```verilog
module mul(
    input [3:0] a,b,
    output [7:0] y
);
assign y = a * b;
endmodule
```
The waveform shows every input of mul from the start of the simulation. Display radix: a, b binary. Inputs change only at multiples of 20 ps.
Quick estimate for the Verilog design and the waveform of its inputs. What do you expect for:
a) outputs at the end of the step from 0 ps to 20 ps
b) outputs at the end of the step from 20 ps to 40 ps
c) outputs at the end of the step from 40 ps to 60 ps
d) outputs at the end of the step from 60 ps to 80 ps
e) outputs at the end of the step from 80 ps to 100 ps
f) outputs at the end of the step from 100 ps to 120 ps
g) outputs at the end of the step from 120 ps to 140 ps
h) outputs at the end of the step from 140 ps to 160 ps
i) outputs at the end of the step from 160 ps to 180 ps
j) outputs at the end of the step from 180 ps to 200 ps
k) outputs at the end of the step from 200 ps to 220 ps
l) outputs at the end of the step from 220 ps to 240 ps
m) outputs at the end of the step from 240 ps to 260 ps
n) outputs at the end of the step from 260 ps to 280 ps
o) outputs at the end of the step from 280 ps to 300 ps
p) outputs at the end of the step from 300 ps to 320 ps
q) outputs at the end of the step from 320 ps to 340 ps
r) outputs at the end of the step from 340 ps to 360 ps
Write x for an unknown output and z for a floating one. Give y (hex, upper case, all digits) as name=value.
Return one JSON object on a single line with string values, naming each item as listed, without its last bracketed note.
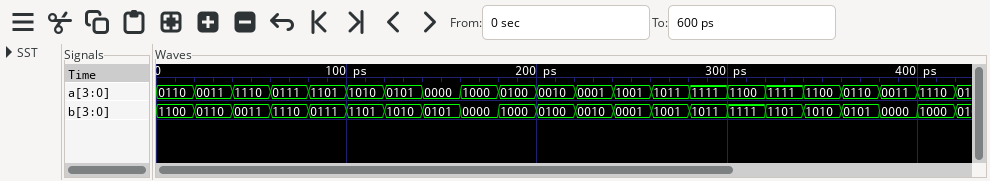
{"outputs at the end of the step from 0 ps to 20 ps": "y=48", "outputs at the end of the step from 20 ps to 40 ps": "y=12", "outputs at the end of the step from 40 ps to 60 ps": "y=2A", "outputs at the end of the step from 60 ps to 80 ps": "y=62", "outputs at the end of the step from 80 ps to 100 ps": "y=5B", "outputs at the end of the step from 100 ps to 120 ps": "y=82", "outputs at the end of the step from 120 ps to 140 ps": "y=32", "outputs at the end of the step from 140 ps to 160 ps": "y=00", "outputs at the end of the step from 160 ps to 180 ps": "y=00", "outputs at the end of the step from 180 ps to 200 ps": "y=20", "outputs at the end of the step from 200 ps to 220 ps": "y=08", "outputs at the end of the step from 220 ps to 240 ps": "y=02", "outputs at the end of the step from 240 ps to 260 ps": "y=09", "outputs at the end of the step from 260 ps to 280 ps": "y=63", "outputs at the end of the step from 280 ps to 300 ps": "y=A5", "outputs at the end of the step from 300 ps to 320 ps": "y=B4", "outputs at the end of the step from 320 ps to 340 ps": "y=C3", "outputs at the end of the step from 340 ps to 360 ps": "y=78"}
